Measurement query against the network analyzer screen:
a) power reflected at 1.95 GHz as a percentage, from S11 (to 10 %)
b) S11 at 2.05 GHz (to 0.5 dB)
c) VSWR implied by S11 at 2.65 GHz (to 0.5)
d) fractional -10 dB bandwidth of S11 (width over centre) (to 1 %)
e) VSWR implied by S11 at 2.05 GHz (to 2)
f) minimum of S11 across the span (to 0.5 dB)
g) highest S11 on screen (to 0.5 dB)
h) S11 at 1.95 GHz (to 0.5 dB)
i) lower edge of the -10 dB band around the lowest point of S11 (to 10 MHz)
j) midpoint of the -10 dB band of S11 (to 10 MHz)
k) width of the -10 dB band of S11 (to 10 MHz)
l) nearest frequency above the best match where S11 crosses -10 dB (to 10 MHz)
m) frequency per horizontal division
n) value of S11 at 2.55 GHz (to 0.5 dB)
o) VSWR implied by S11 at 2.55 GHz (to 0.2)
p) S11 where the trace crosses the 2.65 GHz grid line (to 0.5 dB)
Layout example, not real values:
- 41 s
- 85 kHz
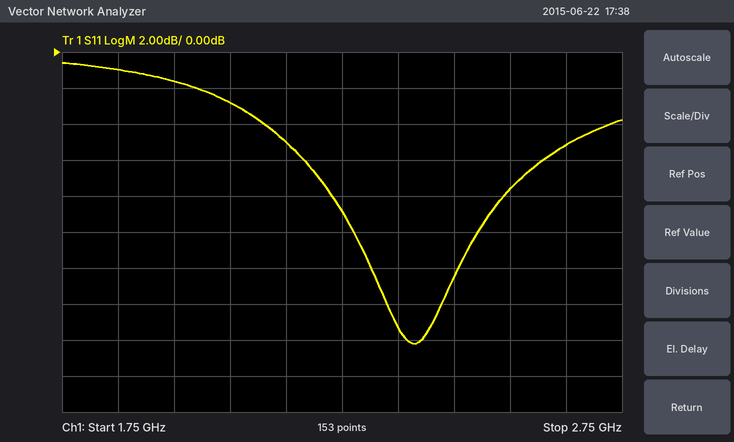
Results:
- 70 %
- -3.0 dB
- 3.5
- 9 %
- 6
- -16.0 dB
- -0.5 dB
- -1.5 dB
- 2.27 GHz
- 2.38 GHz
- 220 MHz
- 2.49 GHz
- 100 MHz
- -7.5 dB
- 2.4
- -5.0 dB
